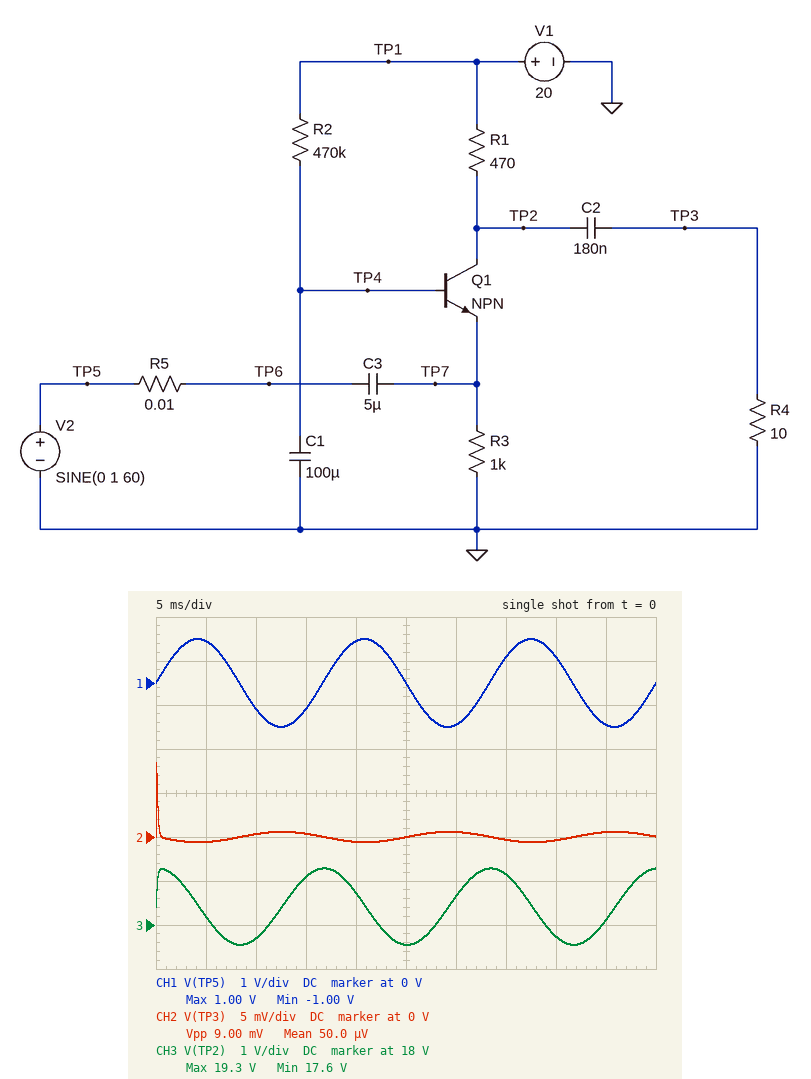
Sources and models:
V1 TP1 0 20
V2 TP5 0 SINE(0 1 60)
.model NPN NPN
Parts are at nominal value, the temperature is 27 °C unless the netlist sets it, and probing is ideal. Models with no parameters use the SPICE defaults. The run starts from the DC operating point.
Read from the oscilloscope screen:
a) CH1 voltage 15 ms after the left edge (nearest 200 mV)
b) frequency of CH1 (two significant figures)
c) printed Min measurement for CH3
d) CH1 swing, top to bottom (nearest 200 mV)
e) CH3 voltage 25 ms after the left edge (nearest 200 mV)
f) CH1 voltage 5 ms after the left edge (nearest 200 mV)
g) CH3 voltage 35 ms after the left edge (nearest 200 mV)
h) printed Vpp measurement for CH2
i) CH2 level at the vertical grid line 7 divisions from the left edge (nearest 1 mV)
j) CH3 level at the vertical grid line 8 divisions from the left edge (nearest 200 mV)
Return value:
-600 mV
60 Hz
17.6 V
2.0 V
17.6 V
1.0 V
19.2 V
9.00 mV
0 V
17.8 V
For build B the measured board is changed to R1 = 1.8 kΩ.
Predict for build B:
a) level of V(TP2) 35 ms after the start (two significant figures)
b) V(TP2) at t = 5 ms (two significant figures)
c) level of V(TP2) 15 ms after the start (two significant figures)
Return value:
17 V
13 V
16 V
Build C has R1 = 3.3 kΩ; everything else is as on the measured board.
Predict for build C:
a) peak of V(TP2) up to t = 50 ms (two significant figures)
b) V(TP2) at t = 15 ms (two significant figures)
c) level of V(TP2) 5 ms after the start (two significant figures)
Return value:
15 V
13 V
8.4 V
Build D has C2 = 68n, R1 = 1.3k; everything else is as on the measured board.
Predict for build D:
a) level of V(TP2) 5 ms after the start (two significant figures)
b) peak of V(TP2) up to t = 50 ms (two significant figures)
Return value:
15 V
18 V
